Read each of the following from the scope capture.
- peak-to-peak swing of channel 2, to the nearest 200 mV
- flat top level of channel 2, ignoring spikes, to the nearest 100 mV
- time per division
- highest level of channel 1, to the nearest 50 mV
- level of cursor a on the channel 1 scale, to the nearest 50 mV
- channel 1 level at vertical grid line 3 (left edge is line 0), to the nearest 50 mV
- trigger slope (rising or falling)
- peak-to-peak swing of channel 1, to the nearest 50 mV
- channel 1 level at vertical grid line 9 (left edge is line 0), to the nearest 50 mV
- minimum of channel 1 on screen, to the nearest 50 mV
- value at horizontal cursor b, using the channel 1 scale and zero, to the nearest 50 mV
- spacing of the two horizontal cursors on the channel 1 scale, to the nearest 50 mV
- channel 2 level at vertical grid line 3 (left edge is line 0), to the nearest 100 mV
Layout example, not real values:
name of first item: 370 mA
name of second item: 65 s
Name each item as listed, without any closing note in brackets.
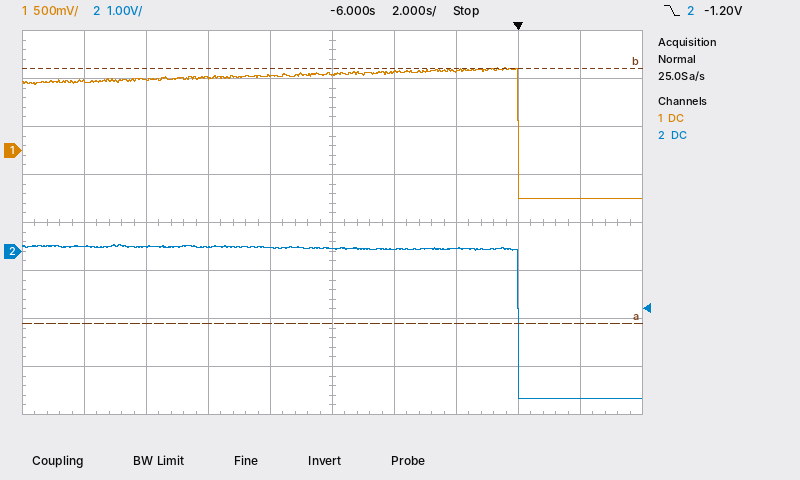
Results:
peak-to-peak swing of channel 2, to the nearest 200 mV: 3.2 V
flat top level of channel 2, ignoring spikes, to the nearest 100 mV: 100 mV
time per division: 2 s
highest level of channel 1, to the nearest 50 mV: 850 mV
level of cursor a on the channel 1 scale, to the nearest 50 mV: -1.80 V
channel 1 level at vertical grid line 3 (left edge is line 0), to the nearest 50 mV: 750 mV
trigger slope: falling
peak-to-peak swing of channel 1, to the nearest 50 mV: 1.35 V
channel 1 level at vertical grid line 9 (left edge is line 0), to the nearest 50 mV: -500 mV
minimum of channel 1 on screen, to the nearest 50 mV: -500 mV
value at horizontal cursor b, using the channel 1 scale and zero, to the nearest 50 mV: 850 mV
spacing of the two horizontal cursors on the channel 1 scale, to the nearest 50 mV: 2.65 V
channel 2 level at vertical grid line 3 (left edge is line 0), to the nearest 100 mV: 100 mV
